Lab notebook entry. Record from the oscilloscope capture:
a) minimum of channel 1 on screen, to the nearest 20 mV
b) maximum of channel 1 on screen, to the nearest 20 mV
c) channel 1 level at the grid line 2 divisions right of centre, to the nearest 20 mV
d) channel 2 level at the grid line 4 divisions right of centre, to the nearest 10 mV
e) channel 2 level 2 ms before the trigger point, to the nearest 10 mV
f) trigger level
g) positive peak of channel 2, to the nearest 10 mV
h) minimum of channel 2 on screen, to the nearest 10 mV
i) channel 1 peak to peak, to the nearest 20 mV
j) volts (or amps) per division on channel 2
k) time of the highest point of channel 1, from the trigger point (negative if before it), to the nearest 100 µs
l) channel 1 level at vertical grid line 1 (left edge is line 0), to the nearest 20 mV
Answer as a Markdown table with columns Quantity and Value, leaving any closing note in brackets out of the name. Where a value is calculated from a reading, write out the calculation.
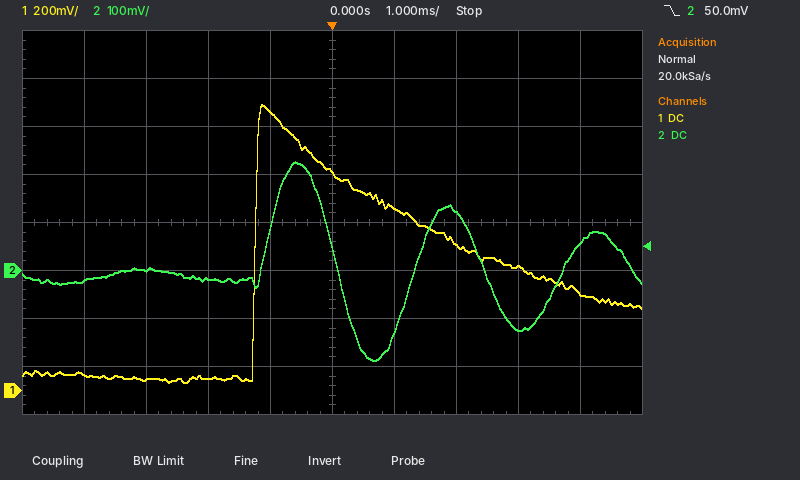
| Quantity | Value |
|---|---|
| minimum of channel 1 on screen, to the nearest 20 mV | 40 mV |
| maximum of channel 1 on screen, to the nearest 20 mV | 1.20 V |
| channel 1 level at the grid line 2 divisions right of centre, to the nearest 20 mV | 600 mV |
| channel 2 level at the grid line 4 divisions right of centre, to the nearest 10 mV | 60 mV |
| channel 2 level 2 ms before the trigger point, to the nearest 10 mV | -20 mV |
| trigger level | 50.0 mV |
| positive peak of channel 2, to the nearest 10 mV | 230 mV |
| minimum of channel 2 on screen, to the nearest 10 mV | -190 mV |
| channel 1 peak to peak, to the nearest 20 mV | 1.20 V − (40 mV) = 1.16 V |
| volts (or amps) per division on channel 2 | 100 mV |
| time of the highest point of channel 1, from the trigger point (negative if before it), to the nearest 100 µs | -1.1 ms |
| channel 1 level at vertical grid line 1 (left edge is line 0), to the nearest 20 mV | 60 mV |
